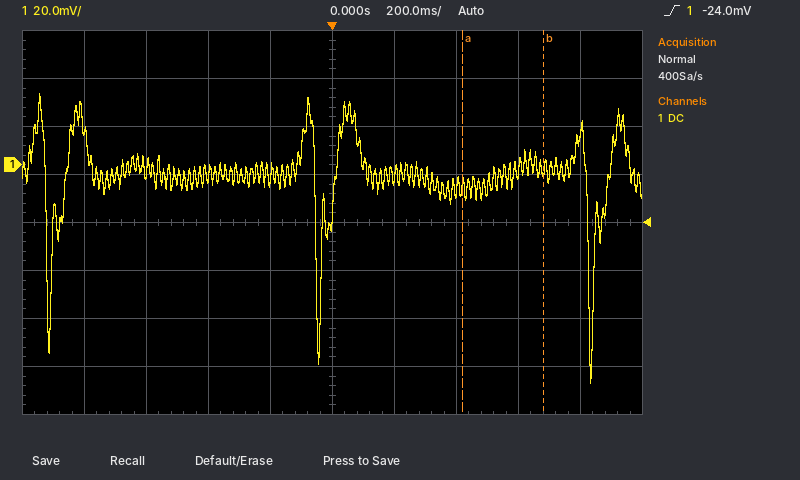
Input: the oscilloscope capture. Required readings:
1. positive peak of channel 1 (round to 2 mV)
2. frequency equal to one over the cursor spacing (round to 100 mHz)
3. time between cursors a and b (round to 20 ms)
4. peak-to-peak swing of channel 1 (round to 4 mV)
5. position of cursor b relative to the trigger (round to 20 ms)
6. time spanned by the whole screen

30 mV
3.8 Hz
260 ms
120 mV
+680 ms
2 s
